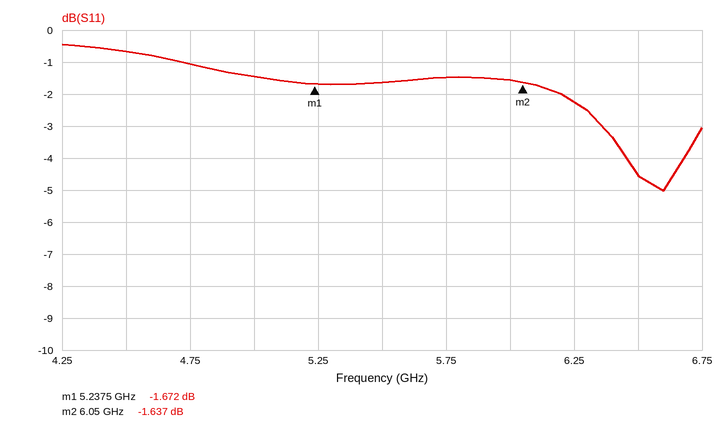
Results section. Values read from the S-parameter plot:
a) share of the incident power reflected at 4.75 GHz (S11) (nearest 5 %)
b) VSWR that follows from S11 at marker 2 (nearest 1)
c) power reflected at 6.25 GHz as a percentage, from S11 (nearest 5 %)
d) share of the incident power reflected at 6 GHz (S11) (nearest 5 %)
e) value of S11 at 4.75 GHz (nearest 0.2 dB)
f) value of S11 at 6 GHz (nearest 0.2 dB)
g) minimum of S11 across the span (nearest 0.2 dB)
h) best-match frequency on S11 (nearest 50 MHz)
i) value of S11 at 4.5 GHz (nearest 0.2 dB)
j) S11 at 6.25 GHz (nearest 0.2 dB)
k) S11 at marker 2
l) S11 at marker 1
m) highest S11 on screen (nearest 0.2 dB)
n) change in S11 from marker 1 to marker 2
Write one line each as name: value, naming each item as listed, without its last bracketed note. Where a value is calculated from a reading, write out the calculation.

share of the incident power reflected at 4.75 GHz (S11): 10^(-1/10) ≈ 79.4 %, so 80 % to the nearest 5 %
VSWR that follows from S11 at marker 2: (1 + 0.8282)/(1 − 0.8282) ≈ 11
power reflected at 6.25 GHz as a percentage, from S11: 10^(-2.2/10) ≈ 60 %
share of the incident power reflected at 6 GHz (S11): 10^(-1.6/10) ≈ 69.2 %, so 70 % to the nearest 5 %
value of S11 at 4.75 GHz: -1.0 dB
value of S11 at 6 GHz: -1.6 dB
minimum of S11 across the span: -5.0 dB
best-match frequency on S11: 6.60 GHz
value of S11 at 4.5 GHz: -0.6 dB
S11 at 6.25 GHz: -2.2 dB
S11 at marker 2: -1.637 dB
S11 at marker 1: -1.672 dB
highest S11 on screen: -0.4 dB
change in S11 from marker 1 to marker 2: -1.637 − (-1.672) = 0.035 dB
